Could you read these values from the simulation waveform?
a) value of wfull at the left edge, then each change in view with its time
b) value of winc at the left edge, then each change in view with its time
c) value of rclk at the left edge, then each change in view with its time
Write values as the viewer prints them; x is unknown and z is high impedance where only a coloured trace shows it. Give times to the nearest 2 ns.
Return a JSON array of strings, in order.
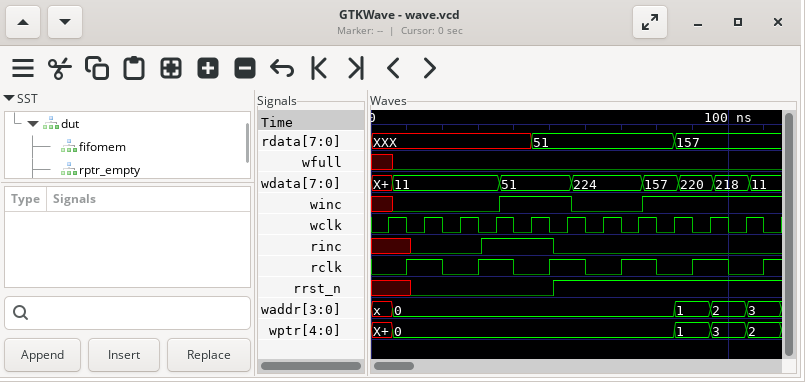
["x, 0 at 6 ns", "x, 0 at 6 ns, 1 at 36 ns, 0 at 56 ns, 1 at 76 ns", "0, 1 at 10 ns, 0 at 20 ns, 1 at 30 ns, 0 at 40 ns, 1 at 50 ns, 0 at 60 ns, 1 at 70 ns, 0 at 80 ns, 1 at 90 ns, 0 at 100 ns, 1 at 110 ns"]
